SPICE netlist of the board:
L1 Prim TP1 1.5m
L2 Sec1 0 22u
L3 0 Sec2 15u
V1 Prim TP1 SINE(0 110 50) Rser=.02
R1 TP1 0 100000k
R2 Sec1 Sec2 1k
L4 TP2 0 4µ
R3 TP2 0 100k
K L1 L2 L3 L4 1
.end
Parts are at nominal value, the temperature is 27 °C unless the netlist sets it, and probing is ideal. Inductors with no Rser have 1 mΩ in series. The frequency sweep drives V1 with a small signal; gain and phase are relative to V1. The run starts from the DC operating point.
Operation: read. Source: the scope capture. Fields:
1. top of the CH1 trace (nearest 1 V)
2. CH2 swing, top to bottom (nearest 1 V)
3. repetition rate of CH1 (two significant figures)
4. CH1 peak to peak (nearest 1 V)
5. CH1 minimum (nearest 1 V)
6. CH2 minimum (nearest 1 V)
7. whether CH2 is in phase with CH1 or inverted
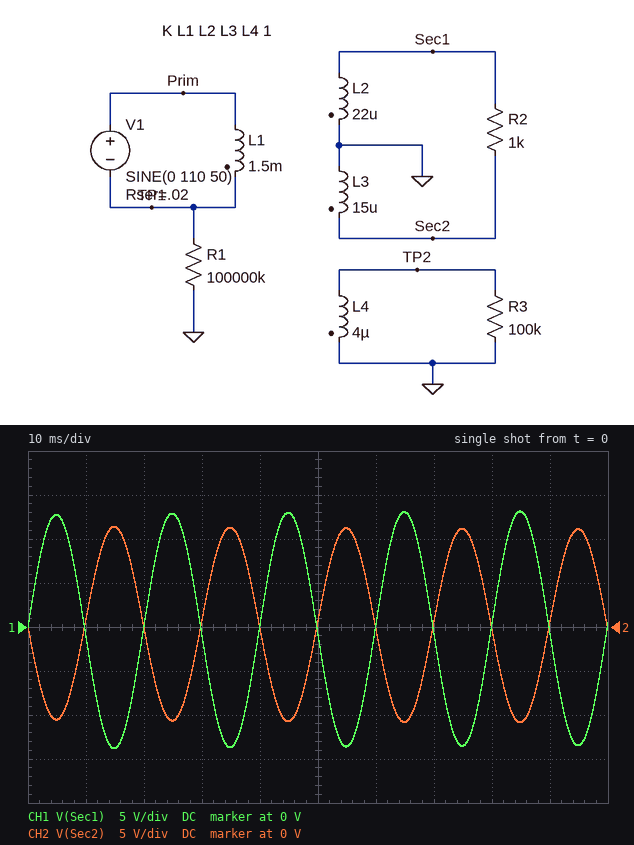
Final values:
13 V
22 V
50 Hz
27 V
-14 V
-11 V
inverted
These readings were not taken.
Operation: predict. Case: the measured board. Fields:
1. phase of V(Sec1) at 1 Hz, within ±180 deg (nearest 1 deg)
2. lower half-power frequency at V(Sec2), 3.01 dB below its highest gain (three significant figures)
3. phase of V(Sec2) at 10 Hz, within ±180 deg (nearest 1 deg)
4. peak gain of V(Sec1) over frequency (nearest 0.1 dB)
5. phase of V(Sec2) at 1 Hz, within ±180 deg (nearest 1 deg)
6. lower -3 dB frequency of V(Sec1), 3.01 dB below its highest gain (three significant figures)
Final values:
66 deg
2.23 Hz
-167 deg
-18.3 dB
-114 deg
2.23 Hz
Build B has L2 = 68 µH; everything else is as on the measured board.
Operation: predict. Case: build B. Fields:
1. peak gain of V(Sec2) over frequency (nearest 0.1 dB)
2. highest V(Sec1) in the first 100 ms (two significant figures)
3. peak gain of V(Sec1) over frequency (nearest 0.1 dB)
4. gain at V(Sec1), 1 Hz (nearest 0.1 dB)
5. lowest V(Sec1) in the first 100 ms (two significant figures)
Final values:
-20.0 dB
23 V
-13.4 dB
-21.2 dB
-24 V
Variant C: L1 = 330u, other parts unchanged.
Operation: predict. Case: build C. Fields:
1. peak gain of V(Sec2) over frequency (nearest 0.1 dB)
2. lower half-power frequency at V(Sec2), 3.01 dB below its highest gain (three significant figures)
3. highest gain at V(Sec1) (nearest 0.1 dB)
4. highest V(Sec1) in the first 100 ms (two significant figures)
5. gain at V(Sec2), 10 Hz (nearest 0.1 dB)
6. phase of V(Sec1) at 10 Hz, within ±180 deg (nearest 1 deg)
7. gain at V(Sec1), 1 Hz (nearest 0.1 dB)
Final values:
-13.4 dB
10.1 Hz
-11.8 dB
28 V
-16.5 dB
45 deg
-31.9 dB
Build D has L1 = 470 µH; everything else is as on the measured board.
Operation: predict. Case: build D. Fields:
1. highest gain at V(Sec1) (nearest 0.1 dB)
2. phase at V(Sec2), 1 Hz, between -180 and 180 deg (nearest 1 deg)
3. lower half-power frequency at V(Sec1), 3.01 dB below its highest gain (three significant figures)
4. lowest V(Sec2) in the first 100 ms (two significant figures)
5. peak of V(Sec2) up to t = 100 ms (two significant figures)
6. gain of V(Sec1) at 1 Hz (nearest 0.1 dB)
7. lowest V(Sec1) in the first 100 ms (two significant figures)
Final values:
-13.3 dB
-98 deg
7.11 Hz
-19 V
21 V
-30.4 dB
-25 V
